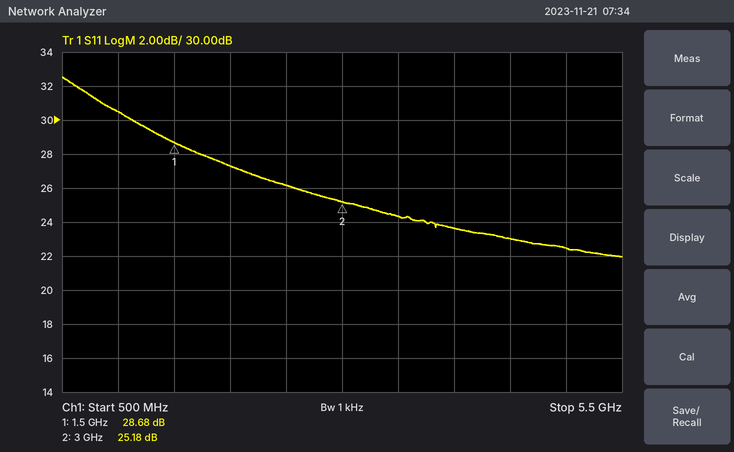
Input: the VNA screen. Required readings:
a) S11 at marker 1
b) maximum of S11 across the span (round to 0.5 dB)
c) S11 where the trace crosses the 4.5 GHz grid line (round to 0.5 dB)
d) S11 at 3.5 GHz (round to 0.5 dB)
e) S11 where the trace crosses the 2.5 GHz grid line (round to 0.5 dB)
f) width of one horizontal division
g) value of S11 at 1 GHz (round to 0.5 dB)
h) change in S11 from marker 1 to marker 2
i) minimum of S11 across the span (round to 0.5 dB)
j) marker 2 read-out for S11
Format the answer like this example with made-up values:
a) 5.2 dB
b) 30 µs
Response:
a) 28.68 dB
b) 32.5 dB
c) 23.0 dB
d) 24.5 dB
e) 26.0 dB
f) 500 MHz
g) 30.5 dB
h) -3.50 dB
i) 22.0 dB
j) 25.18 dB
